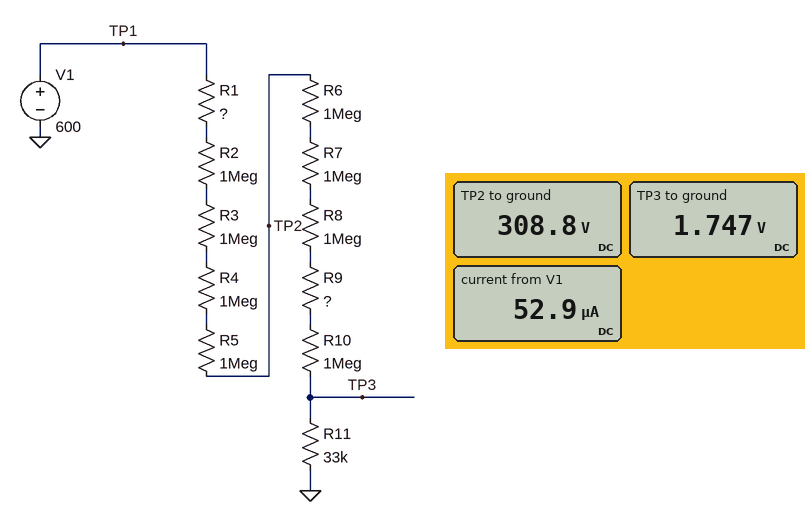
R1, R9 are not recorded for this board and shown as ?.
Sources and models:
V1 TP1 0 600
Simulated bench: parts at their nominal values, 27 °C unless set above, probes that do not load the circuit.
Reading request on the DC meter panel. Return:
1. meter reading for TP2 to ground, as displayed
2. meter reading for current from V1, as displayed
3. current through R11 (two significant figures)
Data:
308.8 V
52.9 µA
53 µA
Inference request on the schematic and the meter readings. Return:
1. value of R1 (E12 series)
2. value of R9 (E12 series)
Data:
1.5 MΩ
1.8 MΩ
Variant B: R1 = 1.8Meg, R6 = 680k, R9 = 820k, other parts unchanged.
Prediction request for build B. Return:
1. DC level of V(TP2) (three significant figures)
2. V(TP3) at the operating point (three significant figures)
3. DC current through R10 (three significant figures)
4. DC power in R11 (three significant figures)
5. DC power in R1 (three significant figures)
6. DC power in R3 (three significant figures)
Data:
263 V
1.92 V
58.1 µA
111 µW
6.07 mW
3.37 mW
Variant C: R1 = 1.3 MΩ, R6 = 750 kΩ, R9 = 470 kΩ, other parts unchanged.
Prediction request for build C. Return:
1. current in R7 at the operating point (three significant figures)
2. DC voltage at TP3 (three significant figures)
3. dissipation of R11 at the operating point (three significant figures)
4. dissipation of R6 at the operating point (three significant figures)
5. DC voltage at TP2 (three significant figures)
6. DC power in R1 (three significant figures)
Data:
62.8 µA
2.07 V
130 µW
2.96 mW
267 V
5.13 mW
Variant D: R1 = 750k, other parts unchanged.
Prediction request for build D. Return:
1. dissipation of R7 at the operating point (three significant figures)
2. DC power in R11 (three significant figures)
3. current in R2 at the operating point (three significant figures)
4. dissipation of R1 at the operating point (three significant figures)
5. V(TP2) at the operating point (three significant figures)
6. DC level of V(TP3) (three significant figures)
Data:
3.21 mW
106 µW
56.7 µA
2.41 mW
331 V
1.87 V
